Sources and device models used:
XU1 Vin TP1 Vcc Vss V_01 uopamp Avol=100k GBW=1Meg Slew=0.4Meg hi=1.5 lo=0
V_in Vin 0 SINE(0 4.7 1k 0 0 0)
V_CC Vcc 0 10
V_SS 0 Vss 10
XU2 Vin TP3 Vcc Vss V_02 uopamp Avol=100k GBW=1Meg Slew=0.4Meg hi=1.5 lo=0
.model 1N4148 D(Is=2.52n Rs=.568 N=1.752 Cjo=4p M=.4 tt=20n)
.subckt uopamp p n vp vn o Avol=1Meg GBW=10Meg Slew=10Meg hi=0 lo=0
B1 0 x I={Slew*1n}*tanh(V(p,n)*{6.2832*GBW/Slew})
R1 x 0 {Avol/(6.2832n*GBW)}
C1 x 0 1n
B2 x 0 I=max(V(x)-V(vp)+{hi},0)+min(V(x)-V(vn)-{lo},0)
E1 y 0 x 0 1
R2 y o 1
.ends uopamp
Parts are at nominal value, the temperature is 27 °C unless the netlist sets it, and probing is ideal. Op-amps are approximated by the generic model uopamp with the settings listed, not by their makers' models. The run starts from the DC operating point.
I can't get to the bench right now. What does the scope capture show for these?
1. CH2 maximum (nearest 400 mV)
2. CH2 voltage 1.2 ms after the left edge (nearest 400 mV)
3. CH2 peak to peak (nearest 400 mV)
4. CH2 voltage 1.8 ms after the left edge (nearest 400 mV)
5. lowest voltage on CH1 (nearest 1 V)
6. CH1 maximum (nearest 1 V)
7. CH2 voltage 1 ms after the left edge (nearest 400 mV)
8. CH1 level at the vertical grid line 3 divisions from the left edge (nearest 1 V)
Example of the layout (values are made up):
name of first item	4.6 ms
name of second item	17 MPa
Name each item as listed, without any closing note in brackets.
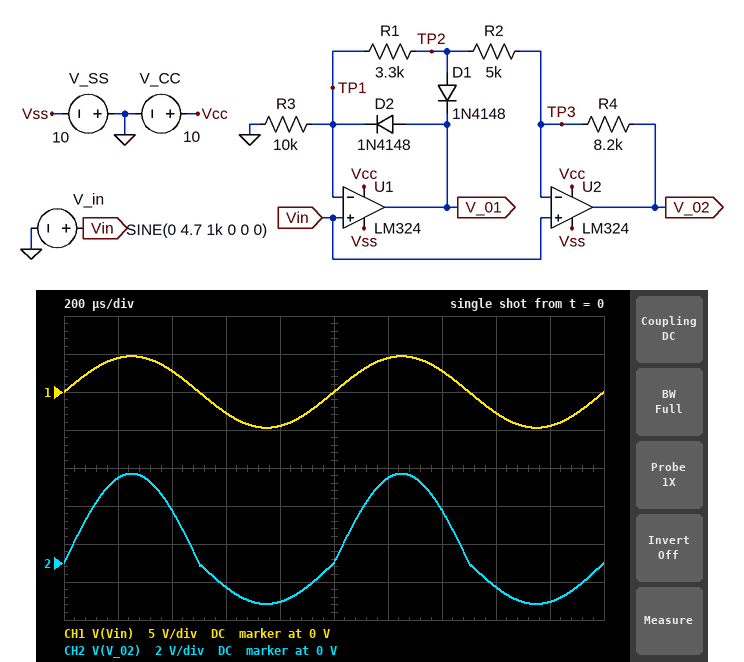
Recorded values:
CH2 maximum	4.8 V
CH2 voltage 1.2 ms after the left edge	4.4 V
CH2 peak to peak	6.8 V
CH2 voltage 1.8 ms after the left edge	-2.0 V
lowest voltage on CH1	-5 V
CH1 maximum	5 V
CH2 voltage 1 ms after the left edge	0 V
CH1 level at the vertical grid line 3 divisions from the left edge	-3 V
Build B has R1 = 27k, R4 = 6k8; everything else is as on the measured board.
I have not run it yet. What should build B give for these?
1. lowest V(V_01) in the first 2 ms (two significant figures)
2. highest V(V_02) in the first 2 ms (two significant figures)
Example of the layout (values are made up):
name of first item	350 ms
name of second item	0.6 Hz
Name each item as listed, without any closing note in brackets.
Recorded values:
lowest V(V_01) in the first 2 ms	-10 V
highest V(V_02) in the first 2 ms	6.8 V
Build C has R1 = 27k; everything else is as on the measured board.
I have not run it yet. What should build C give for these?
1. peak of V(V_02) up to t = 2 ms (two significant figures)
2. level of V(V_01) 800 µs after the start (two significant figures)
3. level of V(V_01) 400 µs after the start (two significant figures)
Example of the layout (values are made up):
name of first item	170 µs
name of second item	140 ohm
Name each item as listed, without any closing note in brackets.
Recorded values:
peak of V(V_02) up to t = 2 ms	8.5 V
level of V(V_01) 800 µs after the start	-10 V
level of V(V_01) 400 µs after the start	3.3 V
